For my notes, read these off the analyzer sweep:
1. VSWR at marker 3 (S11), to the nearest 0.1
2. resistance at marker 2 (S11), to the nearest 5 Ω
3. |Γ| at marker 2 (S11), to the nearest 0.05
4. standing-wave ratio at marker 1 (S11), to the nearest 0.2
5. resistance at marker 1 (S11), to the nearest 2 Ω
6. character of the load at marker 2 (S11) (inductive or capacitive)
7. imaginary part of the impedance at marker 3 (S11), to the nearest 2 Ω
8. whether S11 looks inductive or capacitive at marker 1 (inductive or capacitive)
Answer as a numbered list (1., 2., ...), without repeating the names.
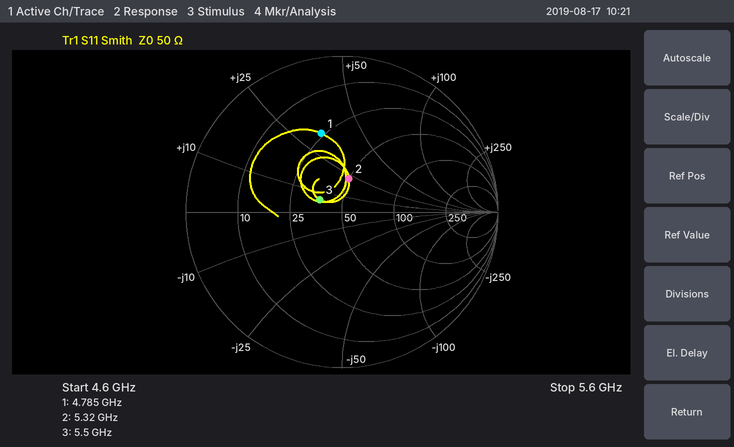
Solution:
1. 1.4
2. 50 Ω
3. 0.20
4. 3.2
5. 24 Ω
6. inductive
7. +6 Ω
8. inductive
